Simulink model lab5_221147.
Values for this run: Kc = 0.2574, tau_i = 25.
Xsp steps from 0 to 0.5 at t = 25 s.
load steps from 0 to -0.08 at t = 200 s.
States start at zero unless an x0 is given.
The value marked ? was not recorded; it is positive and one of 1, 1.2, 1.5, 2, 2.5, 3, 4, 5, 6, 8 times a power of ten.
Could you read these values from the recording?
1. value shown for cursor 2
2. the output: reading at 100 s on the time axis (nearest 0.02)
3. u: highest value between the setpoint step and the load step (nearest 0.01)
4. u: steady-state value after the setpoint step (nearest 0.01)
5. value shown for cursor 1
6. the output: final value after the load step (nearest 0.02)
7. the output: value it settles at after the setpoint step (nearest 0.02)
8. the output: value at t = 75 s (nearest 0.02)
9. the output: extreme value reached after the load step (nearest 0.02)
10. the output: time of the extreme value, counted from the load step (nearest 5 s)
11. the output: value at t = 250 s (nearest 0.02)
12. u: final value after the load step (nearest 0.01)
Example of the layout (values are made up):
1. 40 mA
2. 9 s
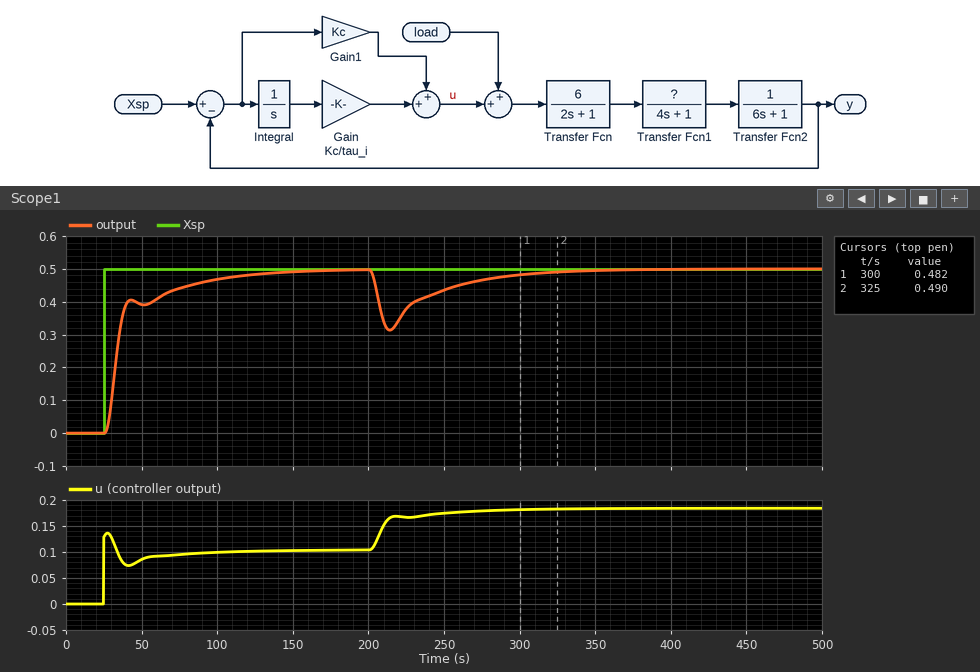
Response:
1. 0.490
2. 0.46
3. 0.14
4. 0.10
5. 0.482
6. 0.50
7. 0.50
8. 0.44
9. 0.32
10. 15 s
11. 0.44
12. 0.18
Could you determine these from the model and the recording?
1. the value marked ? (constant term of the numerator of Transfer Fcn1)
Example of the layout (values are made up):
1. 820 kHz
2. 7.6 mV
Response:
1. 0.8
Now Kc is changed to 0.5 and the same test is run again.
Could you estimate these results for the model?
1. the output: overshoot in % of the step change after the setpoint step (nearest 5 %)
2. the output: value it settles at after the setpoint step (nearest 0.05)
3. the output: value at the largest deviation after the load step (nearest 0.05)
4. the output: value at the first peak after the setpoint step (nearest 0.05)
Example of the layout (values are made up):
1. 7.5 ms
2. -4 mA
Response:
1. 10 %
2. 0.50
3. 0.35
4. 0.55
